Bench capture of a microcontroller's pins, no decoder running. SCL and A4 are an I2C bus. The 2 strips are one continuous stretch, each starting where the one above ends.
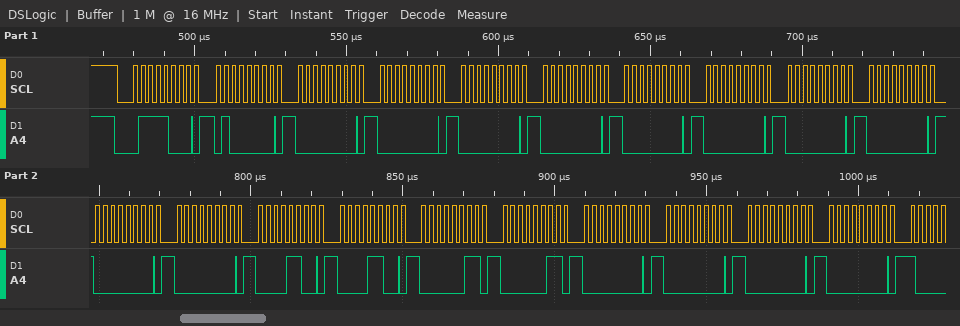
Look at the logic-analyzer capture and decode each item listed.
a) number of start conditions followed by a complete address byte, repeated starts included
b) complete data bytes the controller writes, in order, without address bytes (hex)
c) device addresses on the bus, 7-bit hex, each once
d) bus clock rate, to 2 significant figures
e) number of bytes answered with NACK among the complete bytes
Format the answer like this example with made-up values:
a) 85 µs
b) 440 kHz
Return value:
a) 1
b) 40 00 00 00 00 00 00 00 00 00 00 0C 0C 03 03 00 00 00 00
c) 0x3C
d) 400 kHz
e) 0
